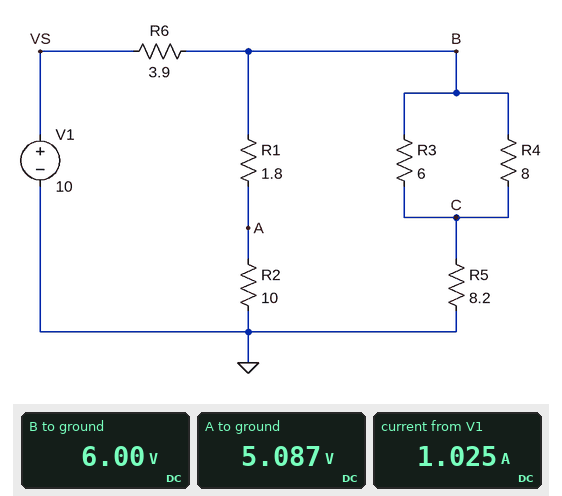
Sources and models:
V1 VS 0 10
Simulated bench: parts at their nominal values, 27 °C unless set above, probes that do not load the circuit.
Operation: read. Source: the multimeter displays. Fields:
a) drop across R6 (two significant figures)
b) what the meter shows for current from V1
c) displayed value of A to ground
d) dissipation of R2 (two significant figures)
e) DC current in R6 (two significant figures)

4.0 V
1.025 A
5.087 V
2.6 W
1.0 A
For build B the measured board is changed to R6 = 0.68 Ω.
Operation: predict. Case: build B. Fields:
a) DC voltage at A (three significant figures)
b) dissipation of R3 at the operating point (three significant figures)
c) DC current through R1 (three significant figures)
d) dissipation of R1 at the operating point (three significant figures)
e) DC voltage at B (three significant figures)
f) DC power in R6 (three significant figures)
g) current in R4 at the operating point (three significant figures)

7.59 V
1.16 W
759 mA
1.04 W
8.96 V
1.59 W
330 mA
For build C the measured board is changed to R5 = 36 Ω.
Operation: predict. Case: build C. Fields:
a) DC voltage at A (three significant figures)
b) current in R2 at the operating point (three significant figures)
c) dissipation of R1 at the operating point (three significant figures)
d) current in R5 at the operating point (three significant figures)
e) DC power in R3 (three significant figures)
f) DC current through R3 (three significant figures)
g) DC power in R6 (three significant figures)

5.93 V
593 mA
633 mW
177 mA
61.7 mW
101 mA
2.31 W
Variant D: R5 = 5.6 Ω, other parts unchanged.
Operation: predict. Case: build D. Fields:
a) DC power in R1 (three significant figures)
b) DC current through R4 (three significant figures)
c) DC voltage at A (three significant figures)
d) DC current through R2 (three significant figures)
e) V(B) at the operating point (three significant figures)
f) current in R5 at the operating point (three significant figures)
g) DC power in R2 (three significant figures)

416 mW
269 mA
4.81 V
481 mA
5.67 V
628 mA
2.31 W
